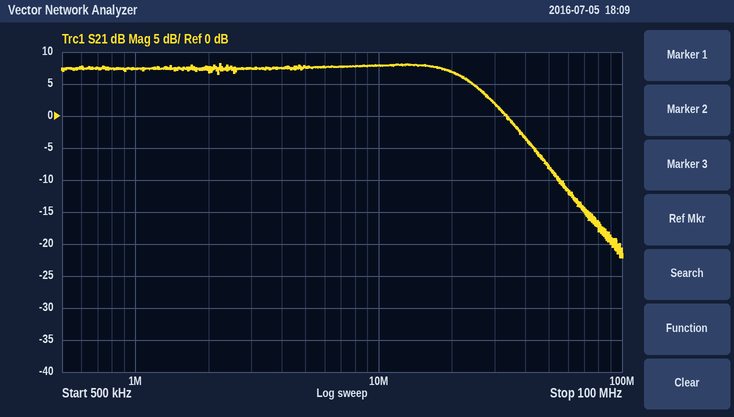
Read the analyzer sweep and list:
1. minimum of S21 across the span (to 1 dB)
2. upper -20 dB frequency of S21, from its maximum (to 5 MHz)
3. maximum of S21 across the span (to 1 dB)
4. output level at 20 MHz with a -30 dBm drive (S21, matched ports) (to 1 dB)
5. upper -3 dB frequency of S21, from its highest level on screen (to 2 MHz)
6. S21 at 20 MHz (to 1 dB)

-22 dB
60 MHz
8 dB
-23 dBm
24 MHz
7 dB
